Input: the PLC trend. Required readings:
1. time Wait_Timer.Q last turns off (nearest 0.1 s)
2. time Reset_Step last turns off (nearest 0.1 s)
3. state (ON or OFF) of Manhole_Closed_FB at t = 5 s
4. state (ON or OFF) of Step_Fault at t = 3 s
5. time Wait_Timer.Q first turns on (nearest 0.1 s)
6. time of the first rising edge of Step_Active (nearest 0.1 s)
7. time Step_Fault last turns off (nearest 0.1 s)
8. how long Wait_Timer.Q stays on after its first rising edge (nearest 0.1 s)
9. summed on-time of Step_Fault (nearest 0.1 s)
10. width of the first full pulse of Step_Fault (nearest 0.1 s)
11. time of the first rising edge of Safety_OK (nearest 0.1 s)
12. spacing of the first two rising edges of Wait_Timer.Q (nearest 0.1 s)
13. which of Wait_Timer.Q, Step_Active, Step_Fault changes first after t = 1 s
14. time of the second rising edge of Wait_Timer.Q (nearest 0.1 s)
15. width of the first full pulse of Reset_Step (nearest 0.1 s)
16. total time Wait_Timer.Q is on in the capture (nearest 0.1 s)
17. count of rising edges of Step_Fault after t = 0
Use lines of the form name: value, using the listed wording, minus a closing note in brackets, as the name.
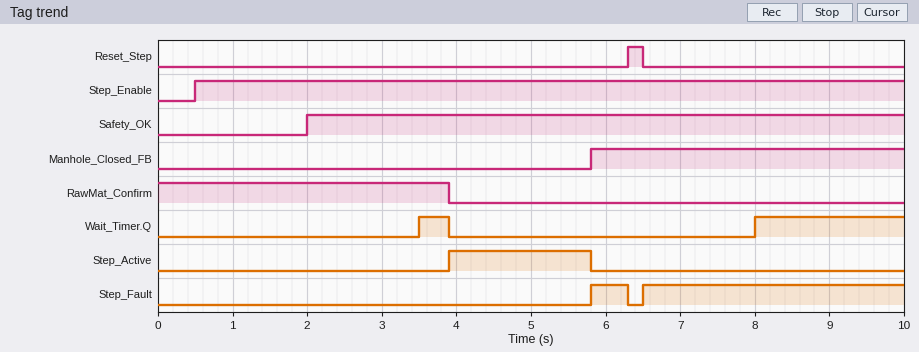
time Wait_Timer.Q last turns off: 3.9 s
time Reset_Step last turns off: 6.5 s
state (ON or OFF) of Manhole_Closed_FB at t = 5 s: OFF
state (ON or OFF) of Step_Fault at t = 3 s: OFF
time Wait_Timer.Q first turns on: 3.5 s
time of the first rising edge of Step_Active: 3.9 s
time Step_Fault last turns off: 6.3 s
how long Wait_Timer.Q stays on after its first rising edge: 0.4 s
summed on-time of Step_Fault: 4.0 s
width of the first full pulse of Step_Fault: 0.5 s
time of the first rising edge of Safety_OK: 2.0 s
spacing of the first two rising edges of Wait_Timer.Q: 4.5 s
which of Wait_Timer.Q, Step_Active, Step_Fault changes first after t = 1 s: Wait_Timer.Q
time of the second rising edge of Wait_Timer.Q: 8.0 s
width of the first full pulse of Reset_Step: 0.2 s
total time Wait_Timer.Q is on in the capture: 2.4 s
count of rising edges of Step_Fault after t = 0: 2
